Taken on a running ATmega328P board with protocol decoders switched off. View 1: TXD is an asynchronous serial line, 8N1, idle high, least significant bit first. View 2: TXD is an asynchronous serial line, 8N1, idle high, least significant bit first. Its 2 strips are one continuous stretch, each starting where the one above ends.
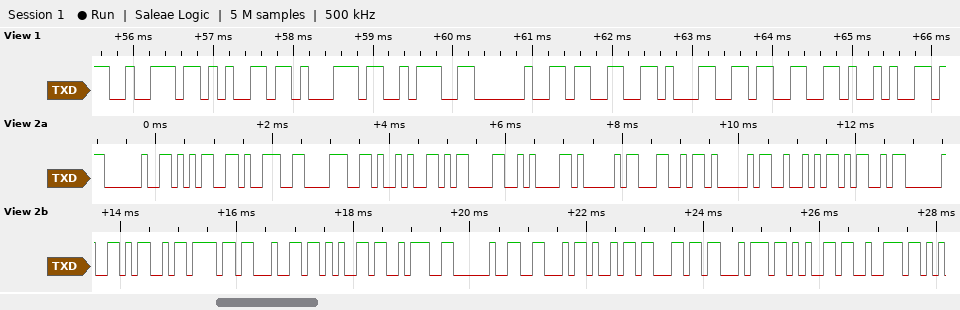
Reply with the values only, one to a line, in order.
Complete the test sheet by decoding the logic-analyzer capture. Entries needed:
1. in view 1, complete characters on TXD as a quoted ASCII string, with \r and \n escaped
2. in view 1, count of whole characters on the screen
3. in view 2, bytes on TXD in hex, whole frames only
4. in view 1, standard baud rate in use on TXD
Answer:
"req: 313)"
9
20 35 39 38 29 0D 0A 41 4C 41 52 4D 20 4D 6F 64 65 3A 20 46 69 6C 74 65 72
9600 baud
